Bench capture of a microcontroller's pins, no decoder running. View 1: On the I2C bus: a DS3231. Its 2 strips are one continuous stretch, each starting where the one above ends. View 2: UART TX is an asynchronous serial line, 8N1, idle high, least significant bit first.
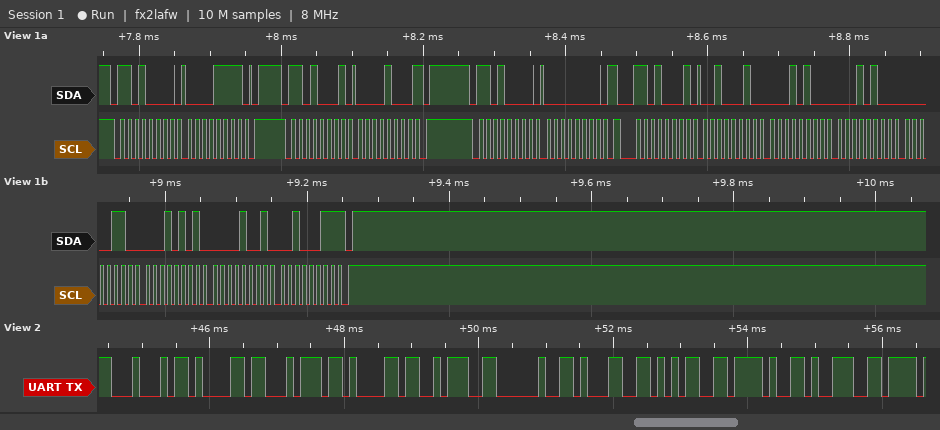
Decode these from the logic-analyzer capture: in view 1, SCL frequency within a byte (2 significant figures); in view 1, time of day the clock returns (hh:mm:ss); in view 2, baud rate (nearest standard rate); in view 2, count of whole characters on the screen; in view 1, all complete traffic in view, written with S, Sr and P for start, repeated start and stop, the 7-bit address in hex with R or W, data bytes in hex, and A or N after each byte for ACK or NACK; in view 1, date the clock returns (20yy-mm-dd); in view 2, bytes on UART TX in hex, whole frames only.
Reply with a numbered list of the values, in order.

1. 100 kHz
2. 14:14:22
3. 9600 baud
4. 10
5. S 68W A 0F A P S 68R A 08 N P S 68W A 00 A Sr 68R A 22 A 14 A 14 A 06 A 15 A 09 A 23 N P
6. 2023-09-15
7. 44 61 74 61 3A 20 31 35 2F 39
